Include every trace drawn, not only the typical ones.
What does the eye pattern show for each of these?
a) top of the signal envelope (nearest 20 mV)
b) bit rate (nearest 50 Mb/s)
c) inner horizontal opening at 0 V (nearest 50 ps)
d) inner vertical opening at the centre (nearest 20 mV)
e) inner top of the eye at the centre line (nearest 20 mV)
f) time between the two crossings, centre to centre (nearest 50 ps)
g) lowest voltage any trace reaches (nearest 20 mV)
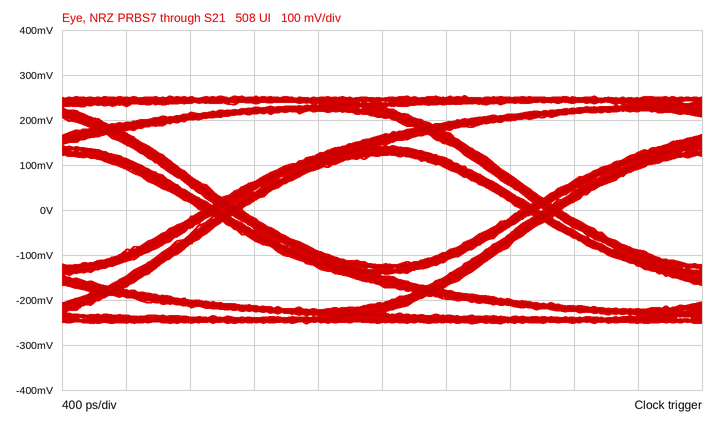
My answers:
260 mV
500 Mb/s
1.75 ns
240 mV
120 mV
2.00 ns
-260 mV
